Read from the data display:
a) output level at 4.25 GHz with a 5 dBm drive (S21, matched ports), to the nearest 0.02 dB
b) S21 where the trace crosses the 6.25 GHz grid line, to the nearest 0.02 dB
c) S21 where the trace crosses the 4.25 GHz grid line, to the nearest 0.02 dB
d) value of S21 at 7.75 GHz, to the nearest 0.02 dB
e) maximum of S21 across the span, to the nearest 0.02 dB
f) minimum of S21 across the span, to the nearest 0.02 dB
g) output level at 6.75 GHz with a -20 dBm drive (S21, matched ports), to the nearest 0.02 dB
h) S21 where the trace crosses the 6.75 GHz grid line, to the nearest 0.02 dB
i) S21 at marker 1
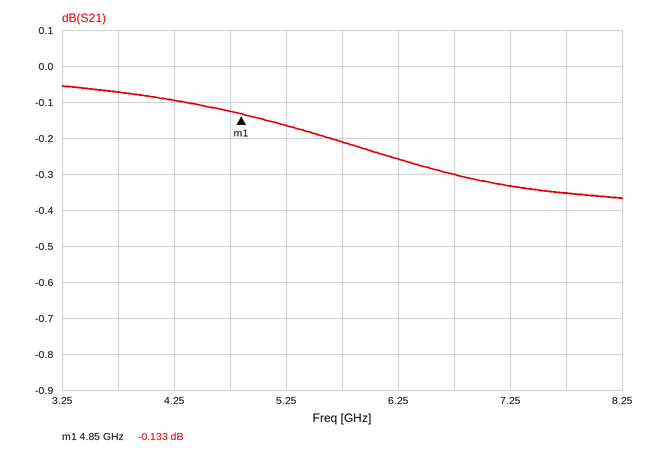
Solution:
4.90 dBm
-0.26 dB
-0.10 dB
-0.36 dB
-0.06 dB
-0.36 dB
-20.30 dBm
-0.30 dB
-0.133 dB
